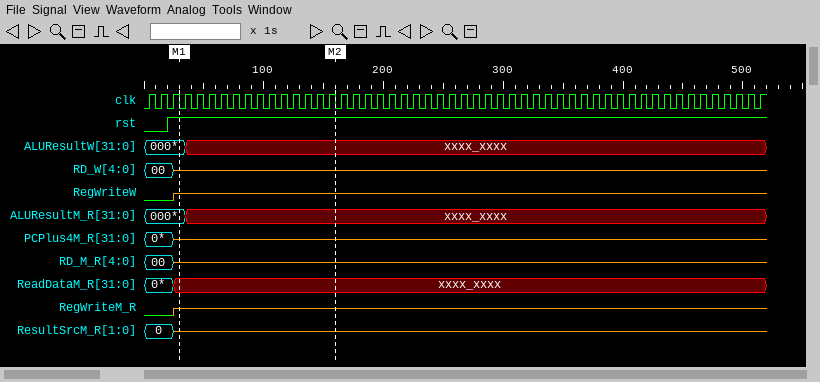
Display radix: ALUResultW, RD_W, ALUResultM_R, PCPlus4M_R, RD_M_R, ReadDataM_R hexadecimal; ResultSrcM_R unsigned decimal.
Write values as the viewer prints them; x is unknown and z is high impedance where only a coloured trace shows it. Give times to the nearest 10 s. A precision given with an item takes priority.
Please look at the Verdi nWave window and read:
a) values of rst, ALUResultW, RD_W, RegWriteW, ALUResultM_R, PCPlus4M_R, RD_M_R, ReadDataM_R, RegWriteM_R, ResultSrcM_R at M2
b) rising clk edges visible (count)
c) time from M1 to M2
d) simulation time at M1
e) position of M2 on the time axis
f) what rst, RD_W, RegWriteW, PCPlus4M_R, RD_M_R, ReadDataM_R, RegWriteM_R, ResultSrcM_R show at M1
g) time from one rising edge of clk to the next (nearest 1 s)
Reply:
rst=1, ALUResultW=xxxx_xxxx, RD_W=z, RegWriteW=z, ALUResultM_R=xxxx_xxxx, PCPlus4M_R=z, RD_M_R=z, ReadDataM_R=xxxx_xxxx, RegWriteM_R=z, ResultSrcM_R=z
52
130 s
30 s
160 s
rst=1, RD_W=z, RegWriteW=z, PCPlus4M_R=z, RD_M_R=z, ReadDataM_R=xxxx_xxxx, RegWriteM_R=z, ResultSrcM_R=z
10 s
